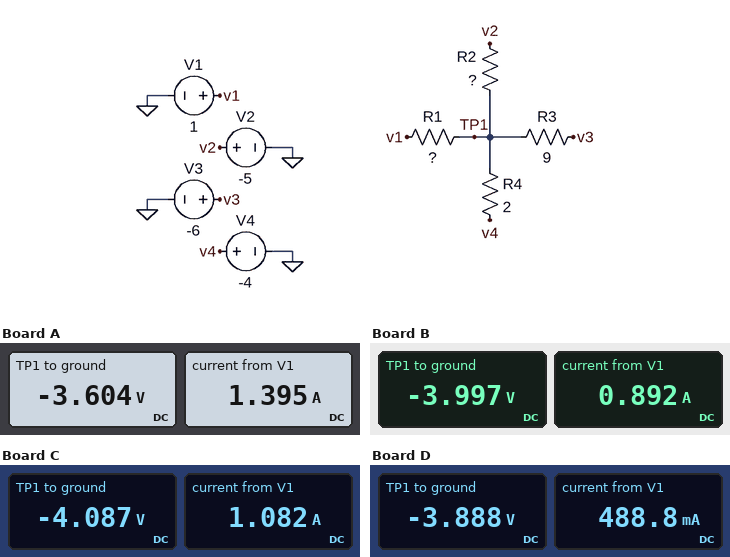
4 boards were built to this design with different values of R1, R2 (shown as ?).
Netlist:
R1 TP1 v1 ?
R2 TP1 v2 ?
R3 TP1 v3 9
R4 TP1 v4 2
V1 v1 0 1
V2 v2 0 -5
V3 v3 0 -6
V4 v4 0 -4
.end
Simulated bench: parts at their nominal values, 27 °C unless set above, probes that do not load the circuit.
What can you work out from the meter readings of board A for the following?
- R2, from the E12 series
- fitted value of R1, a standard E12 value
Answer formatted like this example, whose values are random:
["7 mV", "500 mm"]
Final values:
["1.5 Ω", "3.3 Ω"]
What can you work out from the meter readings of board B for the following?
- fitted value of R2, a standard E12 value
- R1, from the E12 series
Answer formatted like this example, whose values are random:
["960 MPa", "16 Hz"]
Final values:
["1.5 Ω", "5.6 Ω"]
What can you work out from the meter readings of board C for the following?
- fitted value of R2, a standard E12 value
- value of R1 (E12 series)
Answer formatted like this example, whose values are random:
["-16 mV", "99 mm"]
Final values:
["1 Ω", "4.7 Ω"]
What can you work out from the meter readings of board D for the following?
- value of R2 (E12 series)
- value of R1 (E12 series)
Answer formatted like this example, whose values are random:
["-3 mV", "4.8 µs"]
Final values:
["5.6 Ω", "10 Ω"]
